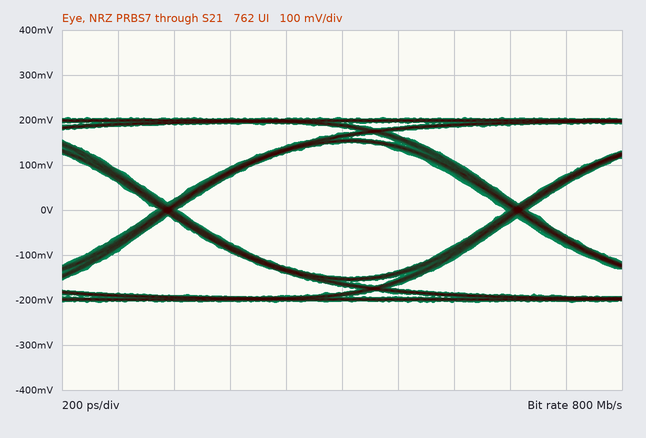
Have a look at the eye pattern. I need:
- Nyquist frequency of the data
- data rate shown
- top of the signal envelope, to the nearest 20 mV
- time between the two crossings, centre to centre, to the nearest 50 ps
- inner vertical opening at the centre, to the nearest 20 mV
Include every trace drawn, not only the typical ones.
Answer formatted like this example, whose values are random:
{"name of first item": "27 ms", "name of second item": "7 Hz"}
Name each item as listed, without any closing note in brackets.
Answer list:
{"Nyquist frequency of the data": "400 MHz", "data rate shown": "800 Mb/s", "top of the signal envelope, to the nearest 20 mV": "200 mV", "time between the two crossings, centre to centre, to the nearest 50 ps": "1.25 ns", "inner vertical opening at the centre, to the nearest 20 mV": "300 mV"}
